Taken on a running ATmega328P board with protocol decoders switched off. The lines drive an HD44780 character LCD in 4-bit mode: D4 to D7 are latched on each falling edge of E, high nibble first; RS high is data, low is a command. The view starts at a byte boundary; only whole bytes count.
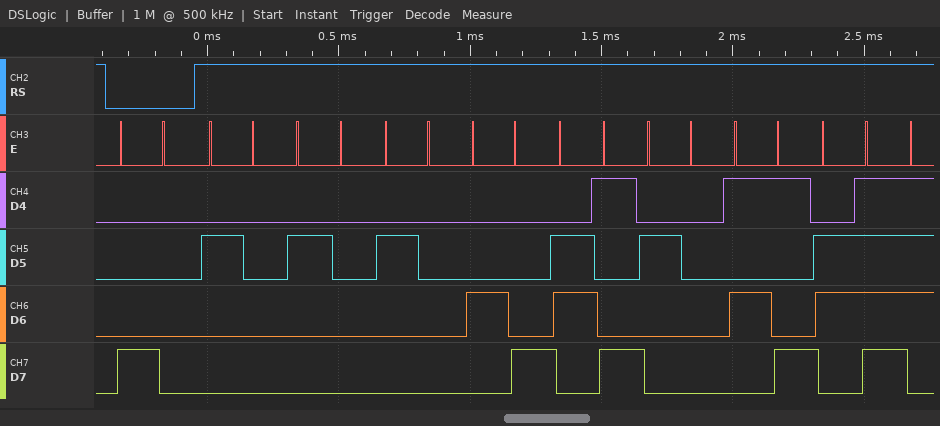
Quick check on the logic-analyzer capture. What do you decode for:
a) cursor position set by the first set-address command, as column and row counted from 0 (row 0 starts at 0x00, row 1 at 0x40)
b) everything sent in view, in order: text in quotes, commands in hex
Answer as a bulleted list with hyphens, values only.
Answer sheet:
- column 0, row 0
- 0x80 "   Hi Yo"
